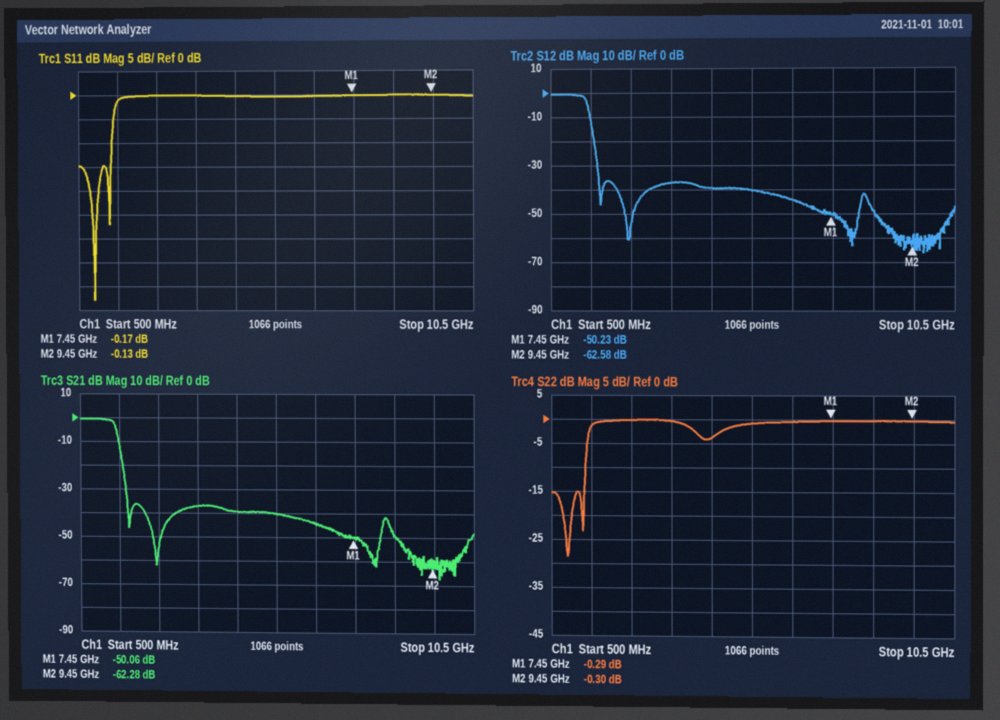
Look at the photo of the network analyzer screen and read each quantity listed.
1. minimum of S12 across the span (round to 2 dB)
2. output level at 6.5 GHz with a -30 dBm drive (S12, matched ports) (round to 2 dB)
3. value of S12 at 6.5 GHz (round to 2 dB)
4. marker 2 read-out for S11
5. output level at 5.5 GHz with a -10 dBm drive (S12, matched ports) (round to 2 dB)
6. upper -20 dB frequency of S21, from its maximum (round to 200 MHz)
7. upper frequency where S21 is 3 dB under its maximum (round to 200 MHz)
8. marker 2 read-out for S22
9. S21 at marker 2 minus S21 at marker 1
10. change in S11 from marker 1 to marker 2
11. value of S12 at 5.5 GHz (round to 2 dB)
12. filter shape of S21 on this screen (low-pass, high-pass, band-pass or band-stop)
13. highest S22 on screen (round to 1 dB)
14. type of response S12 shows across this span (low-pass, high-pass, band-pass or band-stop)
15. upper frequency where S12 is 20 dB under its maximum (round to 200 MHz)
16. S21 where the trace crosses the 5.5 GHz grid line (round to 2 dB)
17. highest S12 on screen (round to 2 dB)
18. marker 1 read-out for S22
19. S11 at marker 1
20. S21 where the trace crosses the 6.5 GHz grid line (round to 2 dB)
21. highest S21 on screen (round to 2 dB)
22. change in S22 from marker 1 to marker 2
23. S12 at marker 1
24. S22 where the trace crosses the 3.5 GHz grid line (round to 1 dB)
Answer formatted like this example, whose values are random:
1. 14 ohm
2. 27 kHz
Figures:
1. -66 dB
2. -74 dBm
3. -44 dB
4. -0.13 dB
5. -50 dBm
6. 1.6 GHz
7. 1.4 GHz
8. -0.30 dB
9. -12.22 dB
10. 0.04 dB
11. -40 dB
12. low-pass
13. 0 dB
14. low-pass
15. 1.6 GHz
16. -40 dB
17. 0 dB
18. -0.29 dB
19. -0.17 dB
20. -44 dB
21. 0 dB
22. -0.01 dB
23. -50.23 dB
24. 0 dB
